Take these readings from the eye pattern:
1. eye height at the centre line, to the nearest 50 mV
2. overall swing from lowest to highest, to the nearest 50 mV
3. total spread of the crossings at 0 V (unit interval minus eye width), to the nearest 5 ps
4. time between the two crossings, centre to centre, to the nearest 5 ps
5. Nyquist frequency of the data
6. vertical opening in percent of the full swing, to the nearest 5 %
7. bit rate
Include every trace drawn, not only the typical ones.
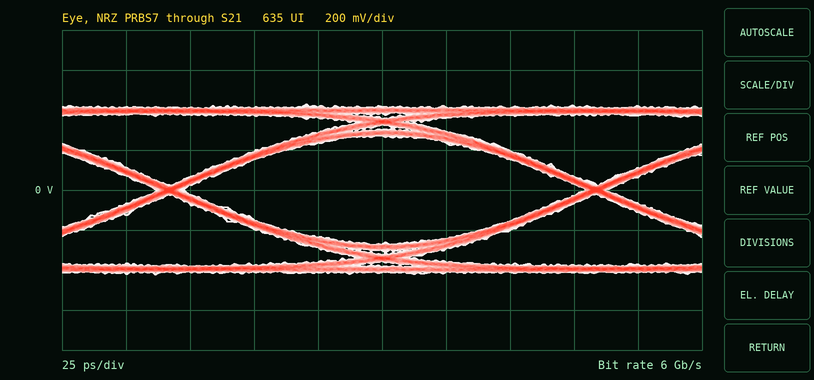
550 mV
850 mV
10 ps
165 ps
3 GHz
65 %
6 Gb/s
